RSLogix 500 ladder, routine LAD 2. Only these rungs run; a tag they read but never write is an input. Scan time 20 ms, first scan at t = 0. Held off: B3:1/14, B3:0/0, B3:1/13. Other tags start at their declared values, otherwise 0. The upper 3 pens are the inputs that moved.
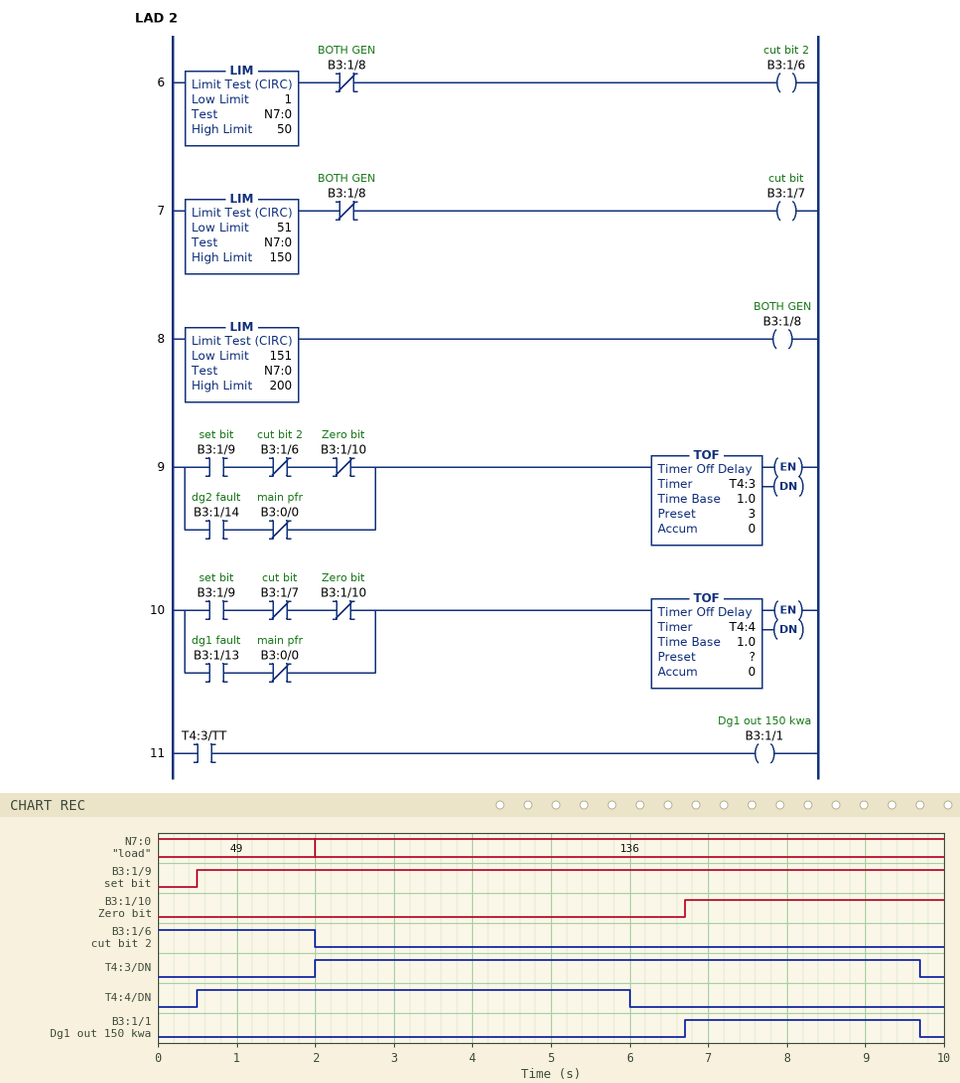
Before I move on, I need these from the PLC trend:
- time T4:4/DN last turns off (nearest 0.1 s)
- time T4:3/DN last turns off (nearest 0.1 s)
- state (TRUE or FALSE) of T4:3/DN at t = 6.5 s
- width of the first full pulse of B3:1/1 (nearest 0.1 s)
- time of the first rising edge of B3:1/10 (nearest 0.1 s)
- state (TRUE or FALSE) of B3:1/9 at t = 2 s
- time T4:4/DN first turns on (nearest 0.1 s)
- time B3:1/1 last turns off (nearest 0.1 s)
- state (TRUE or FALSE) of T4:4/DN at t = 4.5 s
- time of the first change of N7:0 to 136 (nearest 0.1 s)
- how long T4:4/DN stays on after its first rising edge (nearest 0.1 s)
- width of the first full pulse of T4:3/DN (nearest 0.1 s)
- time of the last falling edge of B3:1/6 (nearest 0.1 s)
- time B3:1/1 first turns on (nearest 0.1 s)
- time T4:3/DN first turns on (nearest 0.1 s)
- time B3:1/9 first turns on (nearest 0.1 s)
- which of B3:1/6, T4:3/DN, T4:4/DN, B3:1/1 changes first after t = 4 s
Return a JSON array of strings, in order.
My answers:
["6.0 s", "9.7 s", "TRUE", "3.0 s", "6.7 s", "TRUE", "0.5 s", "9.7 s", "TRUE", "2.0 s", "5.5 s", "7.7 s", "2.0 s", "6.7 s", "2.0 s", "0.5 s", "T4:4/DN"]
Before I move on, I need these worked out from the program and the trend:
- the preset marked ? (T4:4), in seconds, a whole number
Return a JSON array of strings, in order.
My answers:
["4 s"]
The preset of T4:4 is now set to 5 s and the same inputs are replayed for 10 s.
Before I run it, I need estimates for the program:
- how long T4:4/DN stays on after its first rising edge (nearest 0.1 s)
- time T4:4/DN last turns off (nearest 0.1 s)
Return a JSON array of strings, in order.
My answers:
["6.5 s", "7.0 s"]
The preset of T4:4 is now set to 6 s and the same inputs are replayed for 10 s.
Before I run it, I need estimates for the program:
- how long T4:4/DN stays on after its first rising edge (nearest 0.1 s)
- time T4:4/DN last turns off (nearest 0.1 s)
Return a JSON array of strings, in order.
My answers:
["7.5 s", "8.0 s"]
